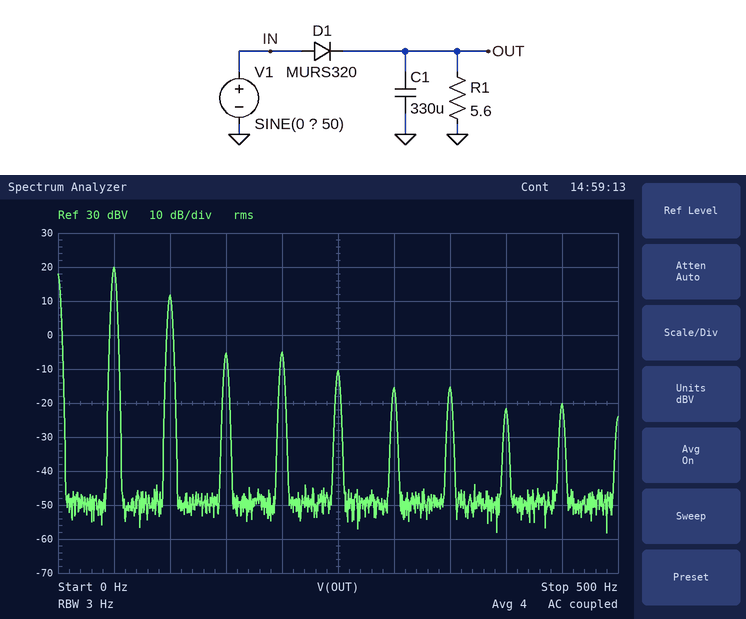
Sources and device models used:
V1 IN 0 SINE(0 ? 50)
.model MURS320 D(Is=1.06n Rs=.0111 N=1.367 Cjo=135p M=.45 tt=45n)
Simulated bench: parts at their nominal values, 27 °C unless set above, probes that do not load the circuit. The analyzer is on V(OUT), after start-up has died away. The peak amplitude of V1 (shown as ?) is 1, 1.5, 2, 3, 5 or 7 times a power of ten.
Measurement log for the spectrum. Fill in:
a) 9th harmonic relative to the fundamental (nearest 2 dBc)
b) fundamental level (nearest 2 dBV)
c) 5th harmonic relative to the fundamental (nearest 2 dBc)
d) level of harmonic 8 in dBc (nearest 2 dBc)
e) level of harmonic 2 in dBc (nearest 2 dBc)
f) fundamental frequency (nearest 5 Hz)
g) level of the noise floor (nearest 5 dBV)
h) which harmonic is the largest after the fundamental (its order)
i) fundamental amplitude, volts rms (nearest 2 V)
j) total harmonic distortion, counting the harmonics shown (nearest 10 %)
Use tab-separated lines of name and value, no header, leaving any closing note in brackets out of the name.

9th harmonic relative to the fundamental	-40 dBc
fundamental level	20 dBV
5th harmonic relative to the fundamental	-30 dBc
level of harmonic 8 in dBc	-42 dBc
level of harmonic 2 in dBc	-8 dBc
fundamental frequency	50 Hz
level of the noise floor	-50 dBV
which harmonic is the largest after the fundamental	2
fundamental amplitude, volts rms	10 V
total harmonic distortion, counting the harmonics shown	40 %
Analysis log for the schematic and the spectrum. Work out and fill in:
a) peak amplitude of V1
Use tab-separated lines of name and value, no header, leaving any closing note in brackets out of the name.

peak amplitude of V1	30 V
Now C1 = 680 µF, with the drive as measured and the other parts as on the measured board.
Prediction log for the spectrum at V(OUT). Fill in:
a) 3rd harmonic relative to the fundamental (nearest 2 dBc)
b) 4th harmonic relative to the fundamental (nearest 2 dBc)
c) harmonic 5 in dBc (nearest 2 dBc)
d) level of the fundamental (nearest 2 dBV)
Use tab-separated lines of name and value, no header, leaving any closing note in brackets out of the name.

3rd harmonic relative to the fundamental	-20 dBc
4th harmonic relative to the fundamental	-28 dBc
harmonic 5 in dBc	-28 dBc
level of the fundamental	20 dBV
